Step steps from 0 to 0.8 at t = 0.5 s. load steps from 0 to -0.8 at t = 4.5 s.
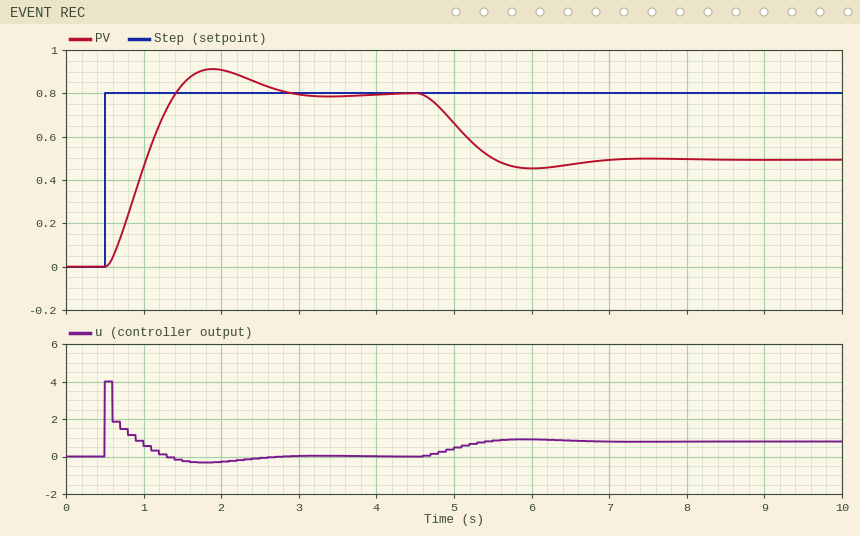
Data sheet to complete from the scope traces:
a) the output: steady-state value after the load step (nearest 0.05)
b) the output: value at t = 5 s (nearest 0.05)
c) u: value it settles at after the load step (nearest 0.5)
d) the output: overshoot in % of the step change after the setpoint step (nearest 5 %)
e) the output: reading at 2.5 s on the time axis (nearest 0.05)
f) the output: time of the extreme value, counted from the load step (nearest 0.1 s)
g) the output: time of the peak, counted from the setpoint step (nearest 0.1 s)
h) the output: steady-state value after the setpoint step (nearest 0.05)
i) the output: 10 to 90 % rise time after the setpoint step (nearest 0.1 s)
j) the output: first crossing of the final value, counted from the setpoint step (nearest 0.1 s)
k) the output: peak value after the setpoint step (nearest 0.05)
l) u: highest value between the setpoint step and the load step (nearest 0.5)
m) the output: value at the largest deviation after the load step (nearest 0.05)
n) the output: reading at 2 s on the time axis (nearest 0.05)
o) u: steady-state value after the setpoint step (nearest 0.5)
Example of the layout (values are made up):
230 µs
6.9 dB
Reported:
0.50
0.65
1.0
15 %
0.85
1.5 s
1.4 s
0.80
0.6 s
0.9 s
0.90
4.0
0.45
0.90
0.0
